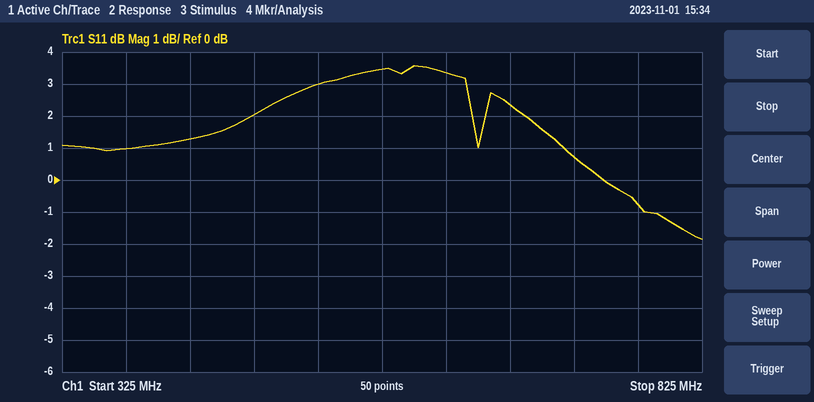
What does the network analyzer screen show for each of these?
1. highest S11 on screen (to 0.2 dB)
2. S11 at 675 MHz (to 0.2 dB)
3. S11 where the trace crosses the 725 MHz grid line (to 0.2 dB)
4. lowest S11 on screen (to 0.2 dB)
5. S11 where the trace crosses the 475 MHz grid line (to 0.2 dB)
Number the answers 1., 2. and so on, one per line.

1. 3.6 dB
2. 2.4 dB
3. 0.8 dB
4. -1.8 dB
5. 2.0 dB
